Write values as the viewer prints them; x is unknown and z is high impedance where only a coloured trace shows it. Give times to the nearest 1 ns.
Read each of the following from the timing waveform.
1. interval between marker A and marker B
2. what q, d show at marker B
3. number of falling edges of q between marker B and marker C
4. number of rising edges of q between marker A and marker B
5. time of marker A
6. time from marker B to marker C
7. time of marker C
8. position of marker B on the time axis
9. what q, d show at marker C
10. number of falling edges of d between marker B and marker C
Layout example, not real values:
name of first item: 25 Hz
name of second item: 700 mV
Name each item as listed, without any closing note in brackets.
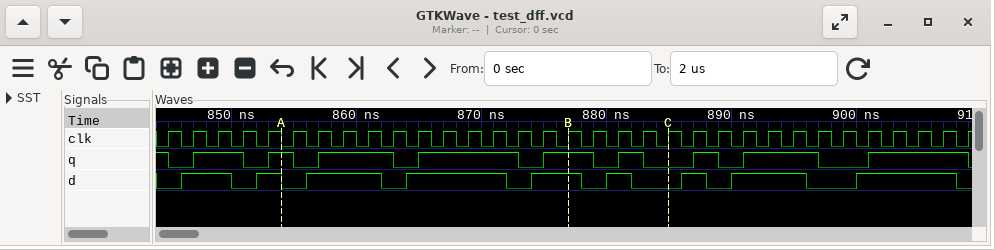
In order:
interval between marker A and marker B: 23 ns
what q, d show at marker B: q=1, d=1
number of falling edges of q between marker B and marker C: 2
number of rising edges of q between marker A and marker B: 3
time of marker A: 854 ns
time from marker B to marker C: 8 ns
time of marker C: 885 ns
position of marker B on the time axis: 877 ns
what q, d show at marker C: q=0, d=0
number of falling edges of d between marker B and marker C: 2
